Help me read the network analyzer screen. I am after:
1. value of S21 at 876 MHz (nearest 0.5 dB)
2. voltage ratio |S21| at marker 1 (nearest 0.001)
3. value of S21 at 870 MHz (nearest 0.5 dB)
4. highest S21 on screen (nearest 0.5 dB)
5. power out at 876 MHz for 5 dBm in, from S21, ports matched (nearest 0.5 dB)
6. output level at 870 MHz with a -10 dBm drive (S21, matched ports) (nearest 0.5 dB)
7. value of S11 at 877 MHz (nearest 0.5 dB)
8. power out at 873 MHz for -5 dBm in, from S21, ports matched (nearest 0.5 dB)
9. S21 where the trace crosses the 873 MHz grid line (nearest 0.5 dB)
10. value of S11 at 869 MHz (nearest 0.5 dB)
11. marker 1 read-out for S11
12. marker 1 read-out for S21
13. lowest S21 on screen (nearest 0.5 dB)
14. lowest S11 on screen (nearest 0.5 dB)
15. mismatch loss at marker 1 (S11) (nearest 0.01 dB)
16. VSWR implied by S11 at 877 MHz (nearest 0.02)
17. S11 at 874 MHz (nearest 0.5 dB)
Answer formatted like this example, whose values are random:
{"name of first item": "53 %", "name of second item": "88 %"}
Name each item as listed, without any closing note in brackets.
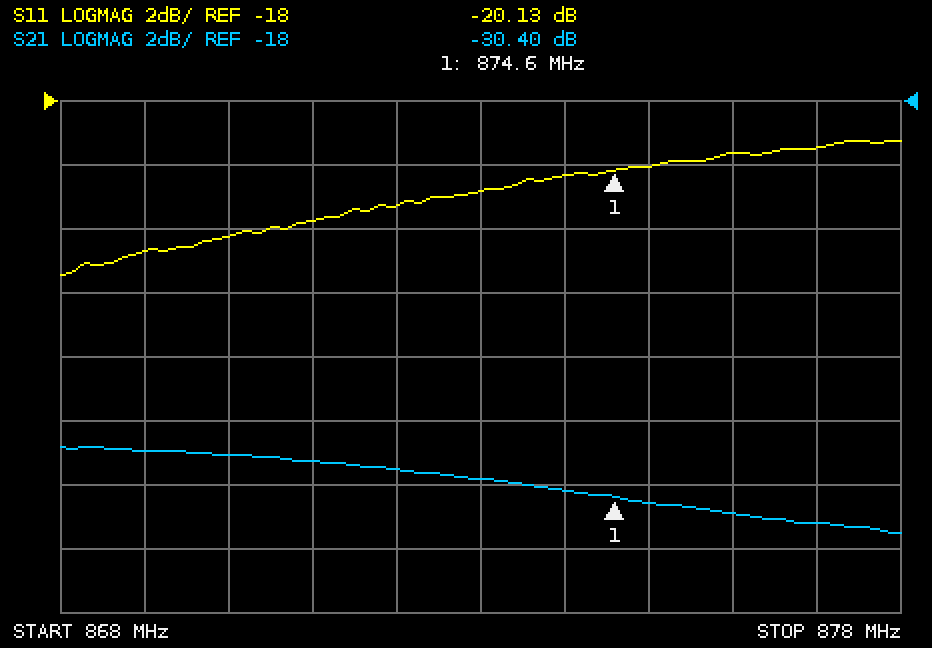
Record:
{"value of S21 at 876 MHz": "-31.0 dB", "voltage ratio |S21| at marker 1": "0.030", "value of S21 at 870 MHz": "-29.0 dB", "highest S21 on screen": "-29.0 dB", "power out at 876 MHz for 5 dBm in, from S21, ports matched": "-26.0 dBm", "output level at 870 MHz with a -10 dBm drive (S21, matched ports)": "-39.0 dBm", "value of S11 at 877 MHz": "-19.5 dB", "power out at 873 MHz for -5 dBm in, from S21, ports matched": "-35.0 dBm", "S21 where the trace crosses the 873 MHz grid line": "-30.0 dB", "value of S11 at 869 MHz": "-22.5 dB", "marker 1 read-out for S11": "-20.13 dB", "marker 1 read-out for S21": "-30.40 dB", "lowest S21 on screen": "-31.5 dB", "lowest S11 on screen": "-23.5 dB", "mismatch loss at marker 1 (S11)": "0.04 dB", "VSWR implied by S11 at 877 MHz": "1.24", "S11 at 874 MHz": "-20.5 dB"}
